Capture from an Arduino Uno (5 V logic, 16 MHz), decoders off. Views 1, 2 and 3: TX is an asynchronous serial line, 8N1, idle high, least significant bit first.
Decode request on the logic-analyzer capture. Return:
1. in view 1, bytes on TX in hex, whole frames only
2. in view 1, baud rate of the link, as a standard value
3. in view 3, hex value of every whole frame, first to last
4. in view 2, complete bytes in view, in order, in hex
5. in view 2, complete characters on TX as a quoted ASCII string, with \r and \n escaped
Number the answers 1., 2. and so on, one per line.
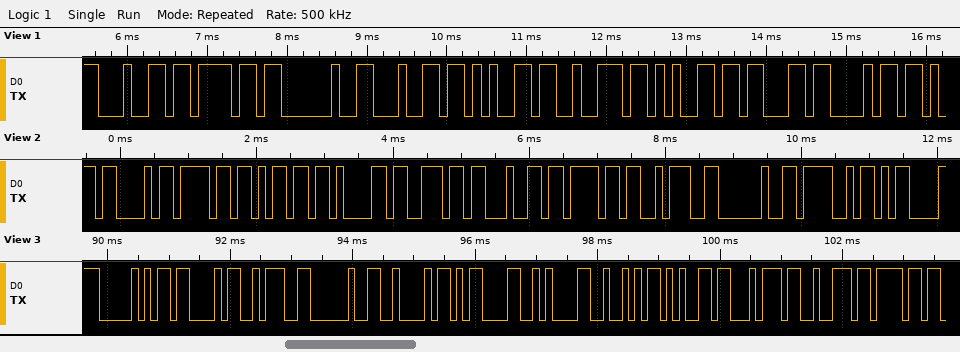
1. 0x64 0x6F 0x20 0x64 0x65 0x72 0x65 0x63 0x68
2. 9600 baud
3. 50 43 3A 20 42 0D 0A 52 65 74 72 6F
4. 43 6F 6D 61 6E 64 6F 3A 20 4F 0D
5. "Comando: O\r"
